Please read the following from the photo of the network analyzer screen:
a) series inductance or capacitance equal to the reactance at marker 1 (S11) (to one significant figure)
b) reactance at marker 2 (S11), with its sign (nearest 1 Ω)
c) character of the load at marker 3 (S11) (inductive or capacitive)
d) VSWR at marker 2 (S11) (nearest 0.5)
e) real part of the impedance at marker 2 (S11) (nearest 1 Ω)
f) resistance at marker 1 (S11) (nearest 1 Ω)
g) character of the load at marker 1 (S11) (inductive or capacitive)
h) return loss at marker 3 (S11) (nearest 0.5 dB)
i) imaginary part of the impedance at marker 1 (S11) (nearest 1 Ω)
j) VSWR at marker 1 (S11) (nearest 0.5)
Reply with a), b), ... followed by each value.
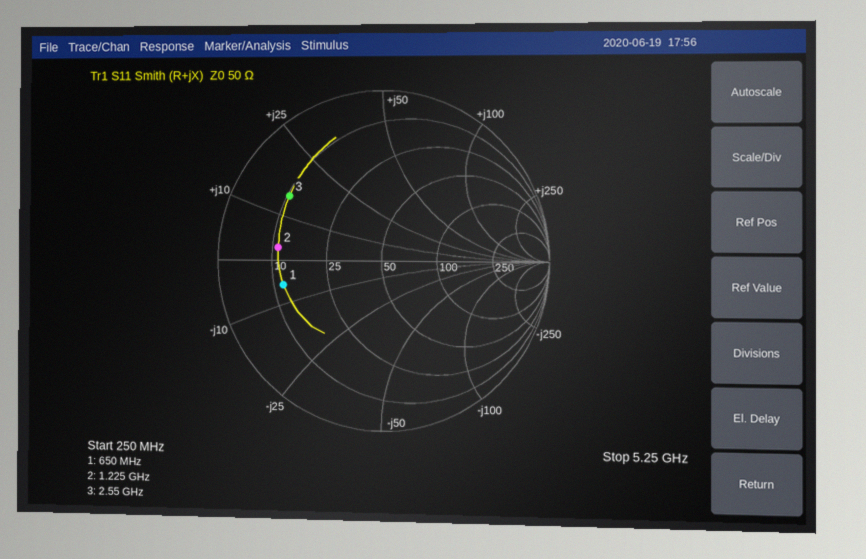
a) 40 pF
b) +3 Ω
c) inductive
d) 4.5
e) 11 Ω
f) 12 Ω
g) capacitive
h) 3.5 dB
i) -6 Ω
j) 4.0
